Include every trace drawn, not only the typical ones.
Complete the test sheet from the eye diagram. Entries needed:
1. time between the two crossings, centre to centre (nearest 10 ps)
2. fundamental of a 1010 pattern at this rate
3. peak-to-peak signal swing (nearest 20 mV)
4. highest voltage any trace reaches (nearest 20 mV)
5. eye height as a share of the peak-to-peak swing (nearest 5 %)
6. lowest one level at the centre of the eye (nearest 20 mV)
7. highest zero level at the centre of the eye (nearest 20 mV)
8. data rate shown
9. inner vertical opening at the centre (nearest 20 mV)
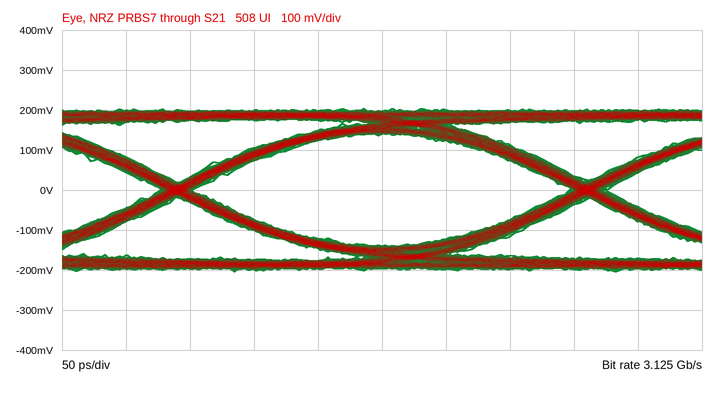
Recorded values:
320 ps
1.5625 GHz
400 mV
200 mV
70 %
140 mV
-140 mV
3.125 Gb/s
280 mV
